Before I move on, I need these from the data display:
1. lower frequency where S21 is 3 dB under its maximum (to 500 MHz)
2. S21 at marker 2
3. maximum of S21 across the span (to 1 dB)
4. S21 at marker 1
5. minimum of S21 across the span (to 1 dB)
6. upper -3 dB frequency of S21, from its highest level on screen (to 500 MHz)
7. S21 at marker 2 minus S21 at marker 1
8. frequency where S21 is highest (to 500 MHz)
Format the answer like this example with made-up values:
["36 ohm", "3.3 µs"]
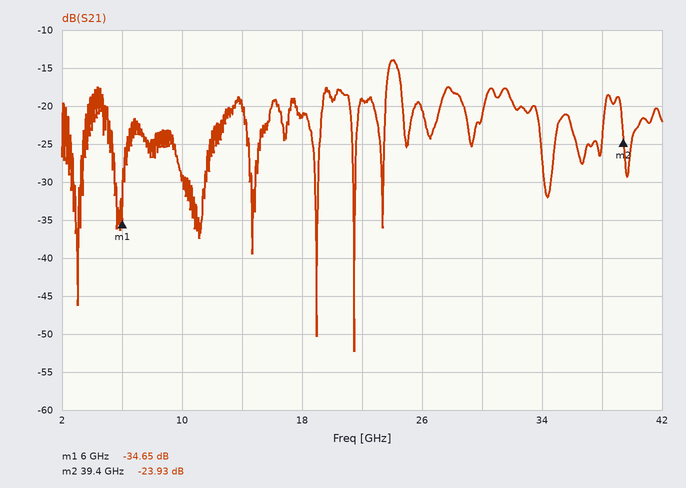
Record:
["23.5 GHz", "-23.93 dB", "-14 dB", "-34.65 dB", "-52 dB", "24.5 GHz", "10.72 dB", "24.0 GHz"]
